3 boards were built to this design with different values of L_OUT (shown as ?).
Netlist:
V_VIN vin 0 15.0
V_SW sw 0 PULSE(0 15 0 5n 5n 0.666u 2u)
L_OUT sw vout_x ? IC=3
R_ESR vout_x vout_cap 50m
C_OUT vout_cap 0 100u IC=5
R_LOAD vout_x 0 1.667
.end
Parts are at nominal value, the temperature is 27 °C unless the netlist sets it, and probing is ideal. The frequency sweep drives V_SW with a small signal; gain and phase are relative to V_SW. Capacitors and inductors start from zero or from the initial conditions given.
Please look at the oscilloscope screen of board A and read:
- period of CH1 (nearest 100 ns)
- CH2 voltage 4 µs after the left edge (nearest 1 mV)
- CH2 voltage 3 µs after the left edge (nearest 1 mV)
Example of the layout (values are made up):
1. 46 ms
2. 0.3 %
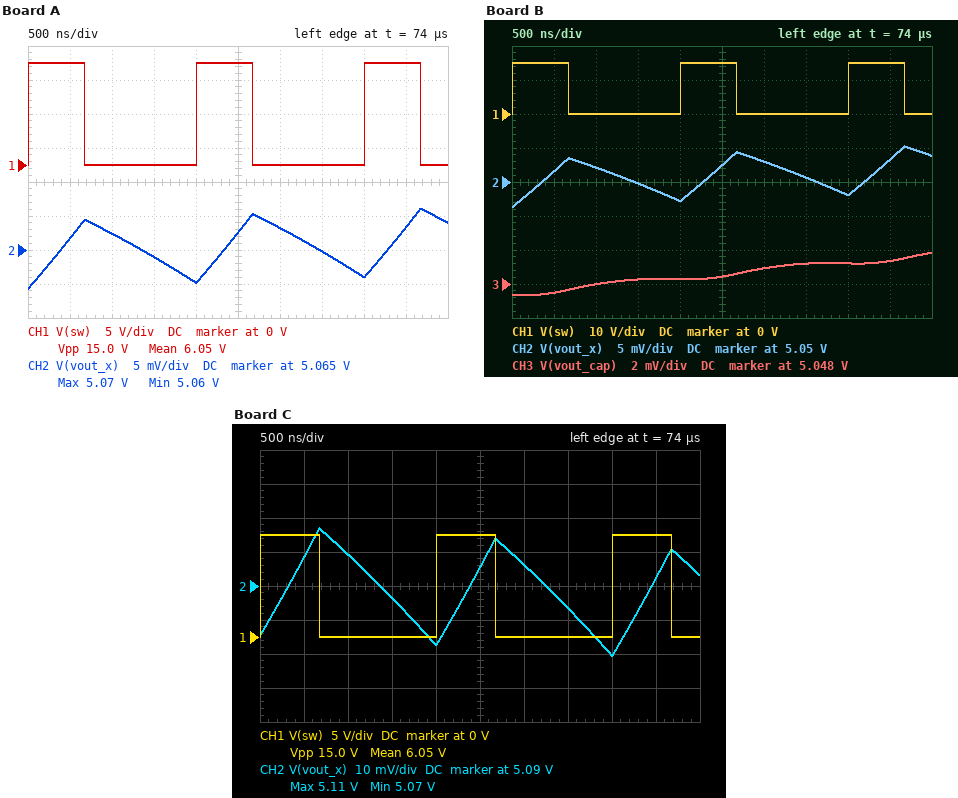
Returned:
1. 2.0 µs
2. 5.061 V
3. 5.068 V
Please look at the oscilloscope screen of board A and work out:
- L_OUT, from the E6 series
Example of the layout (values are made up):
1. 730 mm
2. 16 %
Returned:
1. 33 µH
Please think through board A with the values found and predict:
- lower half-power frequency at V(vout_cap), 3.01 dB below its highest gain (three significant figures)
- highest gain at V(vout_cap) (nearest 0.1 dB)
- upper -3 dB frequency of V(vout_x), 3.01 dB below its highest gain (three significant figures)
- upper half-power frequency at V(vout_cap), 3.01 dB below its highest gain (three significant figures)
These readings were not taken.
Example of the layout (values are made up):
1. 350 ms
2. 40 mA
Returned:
1. 1.92 kHz
2. 7.6 dB
3. 3.14 kHz
4. 3.14 kHz
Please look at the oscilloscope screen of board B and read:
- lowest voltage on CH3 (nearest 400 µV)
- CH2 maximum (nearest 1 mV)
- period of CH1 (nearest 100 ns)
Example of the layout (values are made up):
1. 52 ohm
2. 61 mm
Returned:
1. 5.0472 V
2. 5.055 V
3. 2.0 µs
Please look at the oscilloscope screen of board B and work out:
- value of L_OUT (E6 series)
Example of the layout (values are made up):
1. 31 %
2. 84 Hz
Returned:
1. 47 µH
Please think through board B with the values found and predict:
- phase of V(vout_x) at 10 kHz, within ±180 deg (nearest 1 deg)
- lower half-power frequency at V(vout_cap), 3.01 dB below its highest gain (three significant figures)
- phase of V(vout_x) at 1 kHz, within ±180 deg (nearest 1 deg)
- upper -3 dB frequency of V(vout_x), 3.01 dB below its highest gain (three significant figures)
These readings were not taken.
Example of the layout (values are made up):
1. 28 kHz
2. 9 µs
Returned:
1. -156 deg
2. 1.49 kHz
3. -13 deg
4. 2.66 kHz
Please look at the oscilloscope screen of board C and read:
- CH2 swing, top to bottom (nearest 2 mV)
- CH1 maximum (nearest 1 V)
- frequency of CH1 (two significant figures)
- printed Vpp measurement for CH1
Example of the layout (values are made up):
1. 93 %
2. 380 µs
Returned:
1. 38 mV
2. 15 V
3. 500 kHz
4. 15.0 V
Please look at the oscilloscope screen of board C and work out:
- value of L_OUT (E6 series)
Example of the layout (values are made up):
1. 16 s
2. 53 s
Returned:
1. 10 µH
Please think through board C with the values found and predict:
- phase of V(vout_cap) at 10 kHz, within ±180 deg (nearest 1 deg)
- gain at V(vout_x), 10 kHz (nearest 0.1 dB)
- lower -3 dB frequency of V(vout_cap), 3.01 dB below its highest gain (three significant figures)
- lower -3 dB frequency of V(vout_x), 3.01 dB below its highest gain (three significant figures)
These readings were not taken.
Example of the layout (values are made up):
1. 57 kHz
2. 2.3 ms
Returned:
1. -167 deg
2. -9.5 dB
3. 3.85 kHz
4. 3.86 kHz
